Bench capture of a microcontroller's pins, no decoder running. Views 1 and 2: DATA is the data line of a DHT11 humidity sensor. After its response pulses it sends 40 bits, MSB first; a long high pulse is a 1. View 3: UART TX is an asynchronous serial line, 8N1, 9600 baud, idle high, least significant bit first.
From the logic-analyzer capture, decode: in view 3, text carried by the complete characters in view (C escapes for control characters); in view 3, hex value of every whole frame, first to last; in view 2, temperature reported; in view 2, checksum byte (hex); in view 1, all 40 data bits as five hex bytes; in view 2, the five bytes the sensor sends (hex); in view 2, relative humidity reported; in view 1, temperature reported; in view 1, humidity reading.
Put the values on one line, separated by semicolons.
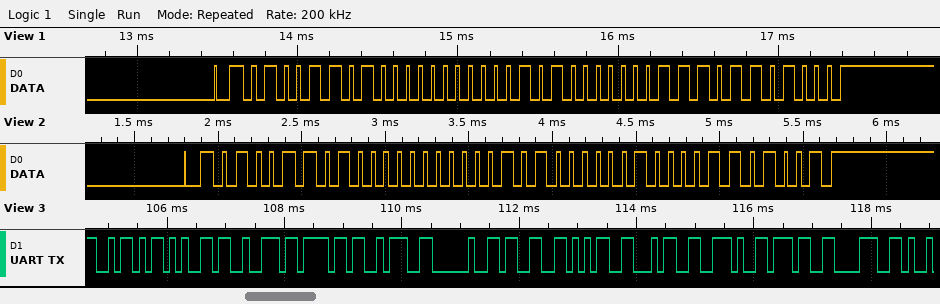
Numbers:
"Zero: 354.78"; 5A 65 72 6F 3A 20 33 35 34 2E 37 38; 20.8 °C; 0x69; 4D 00 14 07 68; 4D 00 14 08 69; 77 %; 20.7 °C; 77 %
